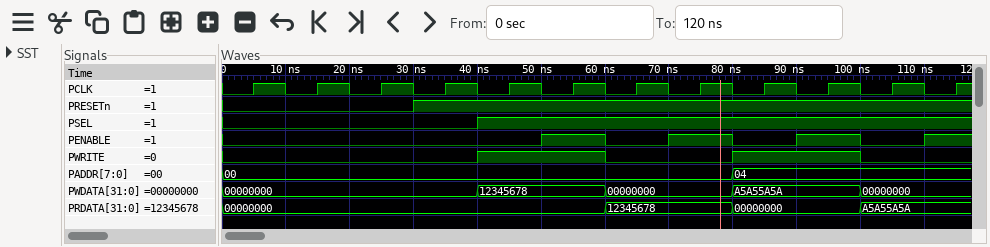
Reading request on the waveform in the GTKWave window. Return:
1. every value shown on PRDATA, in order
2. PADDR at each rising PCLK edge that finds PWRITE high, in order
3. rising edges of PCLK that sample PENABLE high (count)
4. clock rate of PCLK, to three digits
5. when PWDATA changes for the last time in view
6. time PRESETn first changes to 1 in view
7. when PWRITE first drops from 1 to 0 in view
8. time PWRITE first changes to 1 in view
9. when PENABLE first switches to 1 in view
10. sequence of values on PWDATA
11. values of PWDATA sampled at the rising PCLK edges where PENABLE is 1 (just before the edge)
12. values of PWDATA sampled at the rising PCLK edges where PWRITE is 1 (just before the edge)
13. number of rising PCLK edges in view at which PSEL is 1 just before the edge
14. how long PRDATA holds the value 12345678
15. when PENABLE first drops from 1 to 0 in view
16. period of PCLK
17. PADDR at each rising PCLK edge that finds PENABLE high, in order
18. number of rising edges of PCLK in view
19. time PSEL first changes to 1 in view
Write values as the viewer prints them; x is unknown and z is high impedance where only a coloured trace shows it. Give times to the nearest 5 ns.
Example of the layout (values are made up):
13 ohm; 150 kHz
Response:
00000000, 12345678, 00000000, A5A55A5A; 00, 00, 04, 04; 4; 100 MHz; 100 ns; 30 ns; 60 ns; 40 ns; 50 ns; 00000000, 12345678, 00000000, A5A55A5A, 00000000; 12345678, 00000000, A5A55A5A, 00000000; 12345678, 12345678, A5A55A5A, A5A55A5A; 8; 20 ns; 60 ns; 10 ns; 00, 00, 04, 04; 12; 40 ns
